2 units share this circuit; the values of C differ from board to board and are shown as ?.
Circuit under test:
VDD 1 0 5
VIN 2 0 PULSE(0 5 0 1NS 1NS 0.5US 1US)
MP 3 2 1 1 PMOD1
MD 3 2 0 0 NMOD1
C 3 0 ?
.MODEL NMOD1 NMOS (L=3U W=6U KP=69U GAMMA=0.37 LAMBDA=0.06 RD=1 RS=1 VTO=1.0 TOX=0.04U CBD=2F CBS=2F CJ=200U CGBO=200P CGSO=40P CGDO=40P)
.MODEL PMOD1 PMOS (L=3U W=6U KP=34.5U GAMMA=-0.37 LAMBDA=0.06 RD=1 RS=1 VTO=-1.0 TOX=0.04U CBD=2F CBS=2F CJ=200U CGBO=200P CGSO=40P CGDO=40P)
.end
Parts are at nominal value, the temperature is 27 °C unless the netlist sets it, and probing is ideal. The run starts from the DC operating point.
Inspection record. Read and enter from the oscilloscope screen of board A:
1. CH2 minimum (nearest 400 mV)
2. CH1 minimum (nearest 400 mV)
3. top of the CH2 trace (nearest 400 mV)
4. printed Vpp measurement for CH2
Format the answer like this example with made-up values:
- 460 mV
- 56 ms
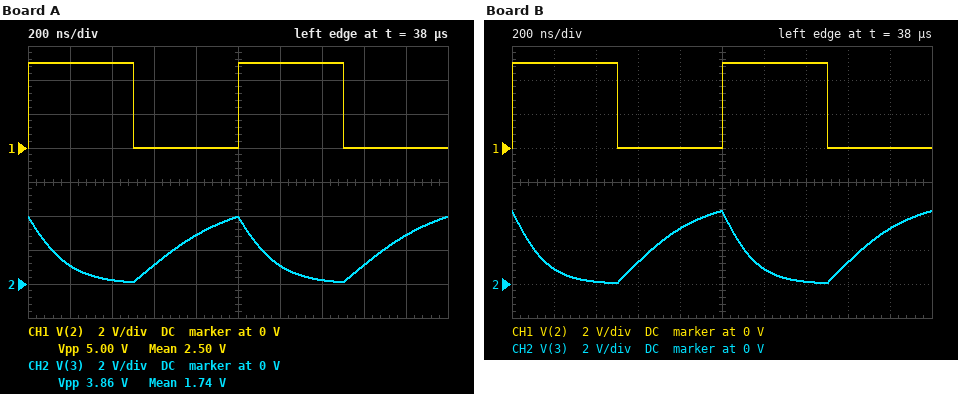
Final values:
- 0 V
- 0 V
- 4.0 V
- 3.86 V
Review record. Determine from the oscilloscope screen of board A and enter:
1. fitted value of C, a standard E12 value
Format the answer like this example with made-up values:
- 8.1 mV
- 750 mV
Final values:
- 68 pF
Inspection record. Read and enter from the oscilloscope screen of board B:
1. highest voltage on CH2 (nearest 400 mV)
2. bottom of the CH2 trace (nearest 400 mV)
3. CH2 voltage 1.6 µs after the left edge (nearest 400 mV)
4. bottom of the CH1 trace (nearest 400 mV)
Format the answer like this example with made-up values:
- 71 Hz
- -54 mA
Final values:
- 4.4 V
- 0 V
- 1.2 V
- 0 V
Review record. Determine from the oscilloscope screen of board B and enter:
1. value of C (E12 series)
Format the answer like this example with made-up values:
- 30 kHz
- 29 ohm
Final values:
- 56 pF
